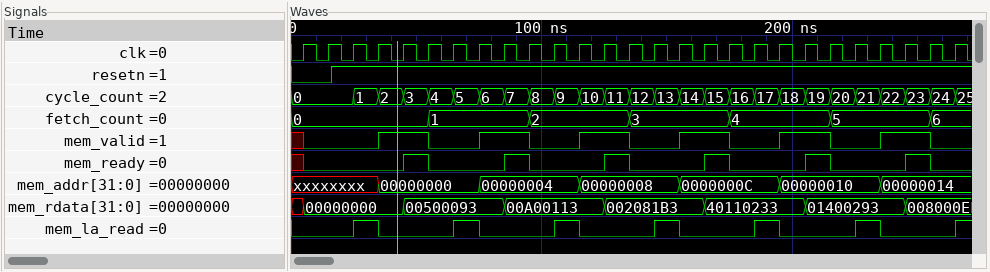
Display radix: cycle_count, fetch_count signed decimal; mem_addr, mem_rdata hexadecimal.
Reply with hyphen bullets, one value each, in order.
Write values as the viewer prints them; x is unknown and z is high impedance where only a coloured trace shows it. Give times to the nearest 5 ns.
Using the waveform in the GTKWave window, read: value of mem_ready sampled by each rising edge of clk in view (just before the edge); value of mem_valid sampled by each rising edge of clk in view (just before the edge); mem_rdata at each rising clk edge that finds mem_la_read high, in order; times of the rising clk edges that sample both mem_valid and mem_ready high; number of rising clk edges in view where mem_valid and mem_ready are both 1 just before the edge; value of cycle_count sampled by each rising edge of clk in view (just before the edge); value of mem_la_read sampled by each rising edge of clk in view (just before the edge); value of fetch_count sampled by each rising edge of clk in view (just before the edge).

- x 0 0 0 0 1 0 0 0 1 0 0 0 1 0 0 0 1 0 0 0 1 0 0 0 1 0
- x 0 0 0 1 1 0 0 1 1 0 0 1 1 0 0 1 1 0 0 1 1 0 0 1 1 0
- 00000000, 00500093, 00A00113, 002081B3, 40110233, 01400293
- 55 ns, 95 ns, 135 ns, 175 ns, 215 ns, 255 ns
- 6
- 0, 0, 0, 1, 2, 3, 4, 5, 6, 7, 8, 9, 10, 11, 12, 13, 14, 15, 16, 17, 18, 19, 20, 21, 22, 23, 24
- 0 0 0 1 0 0 0 1 0 0 0 1 0 0 0 1 0 0 0 1 0 0 0 1 0 0 0
- 0, 0, 0, 0, 0, 0, 1, 1, 1, 1, 2, 2, 2, 2, 3, 3, 3, 3, 4, 4, 4, 4, 5, 5, 5, 5, 6
